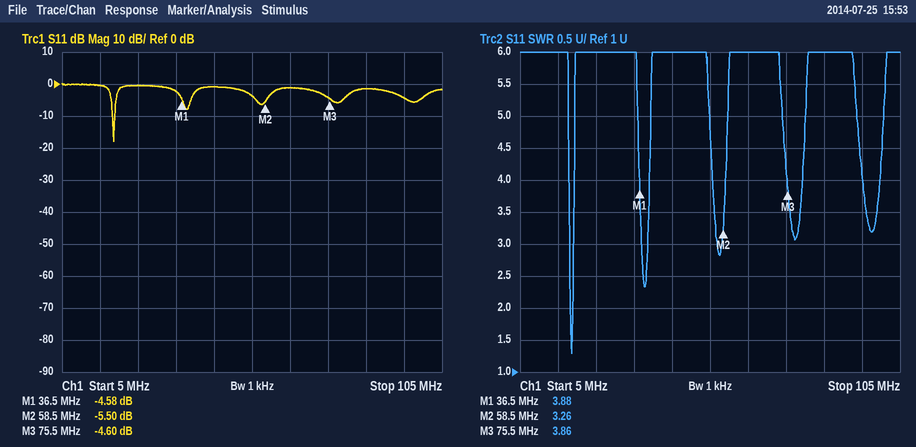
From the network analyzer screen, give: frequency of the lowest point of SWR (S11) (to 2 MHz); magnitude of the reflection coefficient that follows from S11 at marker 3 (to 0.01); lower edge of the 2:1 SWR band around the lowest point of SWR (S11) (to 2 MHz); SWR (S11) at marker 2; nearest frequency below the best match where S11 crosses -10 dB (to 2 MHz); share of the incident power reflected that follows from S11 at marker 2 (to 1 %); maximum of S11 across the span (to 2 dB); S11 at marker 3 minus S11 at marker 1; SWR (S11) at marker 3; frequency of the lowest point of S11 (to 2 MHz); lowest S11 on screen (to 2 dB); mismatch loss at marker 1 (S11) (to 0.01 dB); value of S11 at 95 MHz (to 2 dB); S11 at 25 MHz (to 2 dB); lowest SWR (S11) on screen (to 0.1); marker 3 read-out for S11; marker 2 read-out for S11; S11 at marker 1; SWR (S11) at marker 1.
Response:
18 MHz
0.59
18 MHz
3.26
18 MHz
28 %
0 dB
-0.02 dB
3.86
18 MHz
-18 dB
1.86 dB
-4 dB
0 dB
1.3
-4.60 dB
-5.50 dB
-4.58 dB
3.88
